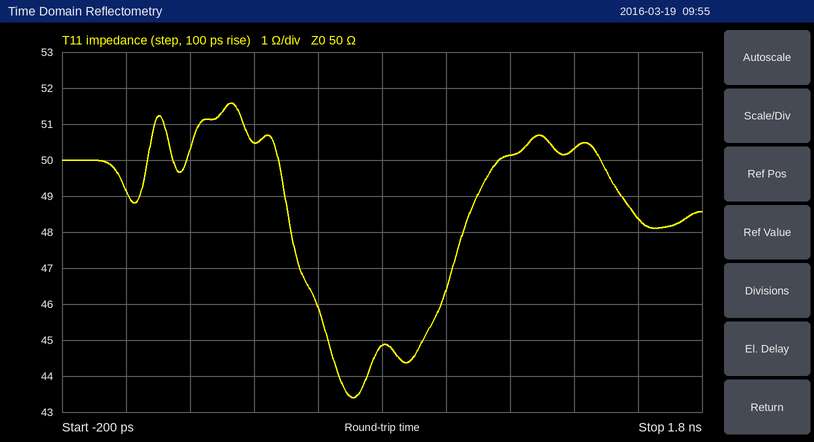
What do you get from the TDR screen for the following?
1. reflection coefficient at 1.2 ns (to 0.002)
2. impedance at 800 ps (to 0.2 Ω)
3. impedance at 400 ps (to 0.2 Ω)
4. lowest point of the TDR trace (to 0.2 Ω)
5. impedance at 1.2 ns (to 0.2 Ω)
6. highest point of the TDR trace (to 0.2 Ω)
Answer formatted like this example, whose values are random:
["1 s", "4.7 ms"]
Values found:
["+0.002", "44.8 Ω", "50.4 Ω", "43.4 Ω", "50.2 Ω", "51.6 Ω"]
